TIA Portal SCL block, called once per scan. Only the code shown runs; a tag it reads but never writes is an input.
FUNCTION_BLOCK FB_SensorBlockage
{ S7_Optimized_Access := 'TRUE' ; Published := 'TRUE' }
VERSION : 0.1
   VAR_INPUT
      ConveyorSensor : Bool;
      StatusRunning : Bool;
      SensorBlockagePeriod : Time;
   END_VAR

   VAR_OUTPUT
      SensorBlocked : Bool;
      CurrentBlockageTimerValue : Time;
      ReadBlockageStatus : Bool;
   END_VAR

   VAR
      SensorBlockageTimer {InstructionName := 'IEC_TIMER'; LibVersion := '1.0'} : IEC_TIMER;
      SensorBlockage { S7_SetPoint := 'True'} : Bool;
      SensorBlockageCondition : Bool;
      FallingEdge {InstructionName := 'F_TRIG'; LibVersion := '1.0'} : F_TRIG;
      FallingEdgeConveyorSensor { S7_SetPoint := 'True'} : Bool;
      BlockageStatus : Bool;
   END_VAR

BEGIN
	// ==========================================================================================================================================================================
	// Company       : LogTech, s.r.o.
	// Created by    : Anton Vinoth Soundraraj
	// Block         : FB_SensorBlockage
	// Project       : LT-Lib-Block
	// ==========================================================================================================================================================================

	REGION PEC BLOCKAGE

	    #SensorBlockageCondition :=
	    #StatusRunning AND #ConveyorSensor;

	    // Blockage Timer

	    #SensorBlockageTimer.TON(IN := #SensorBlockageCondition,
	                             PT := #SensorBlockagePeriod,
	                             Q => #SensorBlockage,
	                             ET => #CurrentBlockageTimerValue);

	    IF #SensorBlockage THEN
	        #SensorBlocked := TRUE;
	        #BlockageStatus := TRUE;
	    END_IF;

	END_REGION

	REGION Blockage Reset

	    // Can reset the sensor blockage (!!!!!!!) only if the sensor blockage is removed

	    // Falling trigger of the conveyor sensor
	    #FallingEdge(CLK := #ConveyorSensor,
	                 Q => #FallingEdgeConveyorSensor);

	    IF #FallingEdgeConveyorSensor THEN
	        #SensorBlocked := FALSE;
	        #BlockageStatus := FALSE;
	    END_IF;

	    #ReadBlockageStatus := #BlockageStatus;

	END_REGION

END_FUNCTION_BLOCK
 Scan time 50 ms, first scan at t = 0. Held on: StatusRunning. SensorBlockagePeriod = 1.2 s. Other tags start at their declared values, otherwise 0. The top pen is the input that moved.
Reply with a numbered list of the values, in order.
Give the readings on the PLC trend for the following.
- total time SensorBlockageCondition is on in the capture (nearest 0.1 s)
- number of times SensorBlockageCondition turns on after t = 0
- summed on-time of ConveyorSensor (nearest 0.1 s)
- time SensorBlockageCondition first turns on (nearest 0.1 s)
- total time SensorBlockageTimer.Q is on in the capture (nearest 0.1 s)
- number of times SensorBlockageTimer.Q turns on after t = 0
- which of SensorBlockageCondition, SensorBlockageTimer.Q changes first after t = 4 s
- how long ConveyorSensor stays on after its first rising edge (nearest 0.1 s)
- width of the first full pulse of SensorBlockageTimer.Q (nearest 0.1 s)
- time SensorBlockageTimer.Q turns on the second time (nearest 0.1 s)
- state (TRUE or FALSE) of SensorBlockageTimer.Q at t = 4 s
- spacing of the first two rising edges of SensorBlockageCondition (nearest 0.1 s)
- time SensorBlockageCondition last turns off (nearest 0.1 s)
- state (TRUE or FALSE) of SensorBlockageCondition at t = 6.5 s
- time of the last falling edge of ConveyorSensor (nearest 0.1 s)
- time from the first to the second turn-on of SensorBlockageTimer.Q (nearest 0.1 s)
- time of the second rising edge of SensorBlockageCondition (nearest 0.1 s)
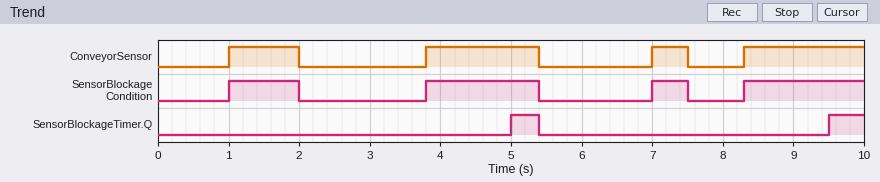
1. 4.8 s
2. 4
3. 4.8 s
4. 1.0 s
5. 0.9 s
6. 2
7. SensorBlockageTimer.Q
8. 1.0 s
9. 0.4 s
10. 9.5 s
11. FALSE
12. 2.8 s
13. 7.5 s
14. FALSE
15. 7.5 s
16. 4.5 s
17. 3.8 s
